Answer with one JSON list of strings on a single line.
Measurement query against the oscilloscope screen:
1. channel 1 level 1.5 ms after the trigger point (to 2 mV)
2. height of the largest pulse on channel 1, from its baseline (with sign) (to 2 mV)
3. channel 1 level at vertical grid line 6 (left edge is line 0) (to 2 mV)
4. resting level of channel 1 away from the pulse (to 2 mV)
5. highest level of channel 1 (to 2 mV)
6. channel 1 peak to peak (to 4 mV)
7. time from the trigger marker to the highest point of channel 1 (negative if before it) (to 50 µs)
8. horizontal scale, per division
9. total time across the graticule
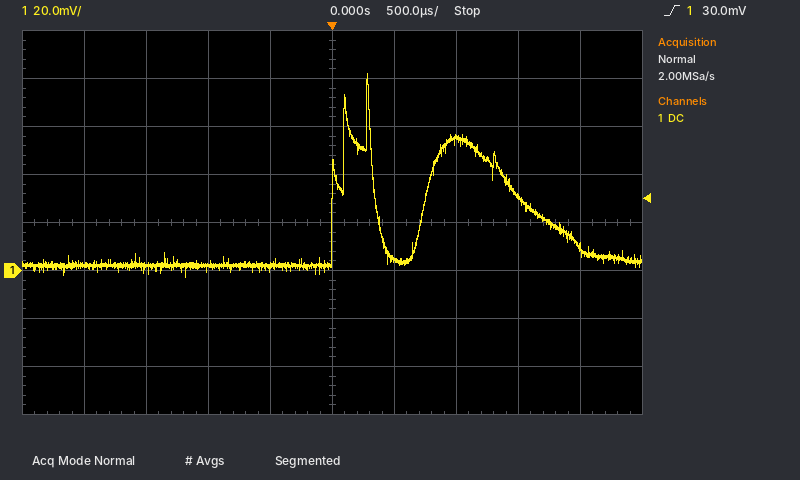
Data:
["30 mV", "+80 mV", "4 mV", "2 mV", "82 mV", "84 mV", "+300 µs", "500 µs", "5 ms"]
